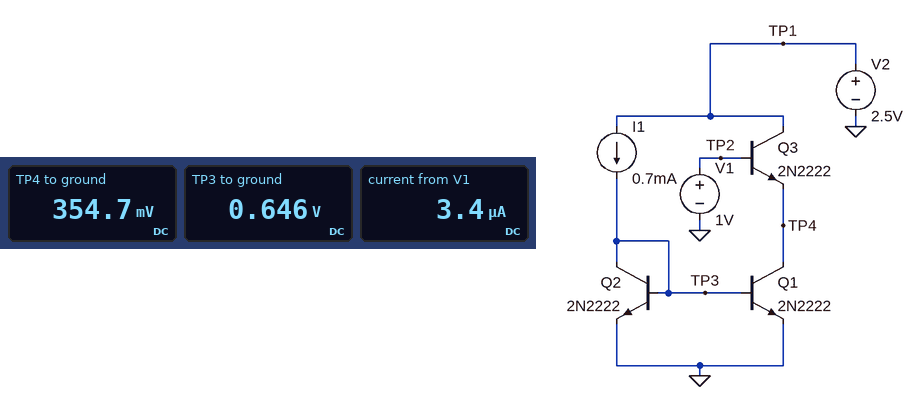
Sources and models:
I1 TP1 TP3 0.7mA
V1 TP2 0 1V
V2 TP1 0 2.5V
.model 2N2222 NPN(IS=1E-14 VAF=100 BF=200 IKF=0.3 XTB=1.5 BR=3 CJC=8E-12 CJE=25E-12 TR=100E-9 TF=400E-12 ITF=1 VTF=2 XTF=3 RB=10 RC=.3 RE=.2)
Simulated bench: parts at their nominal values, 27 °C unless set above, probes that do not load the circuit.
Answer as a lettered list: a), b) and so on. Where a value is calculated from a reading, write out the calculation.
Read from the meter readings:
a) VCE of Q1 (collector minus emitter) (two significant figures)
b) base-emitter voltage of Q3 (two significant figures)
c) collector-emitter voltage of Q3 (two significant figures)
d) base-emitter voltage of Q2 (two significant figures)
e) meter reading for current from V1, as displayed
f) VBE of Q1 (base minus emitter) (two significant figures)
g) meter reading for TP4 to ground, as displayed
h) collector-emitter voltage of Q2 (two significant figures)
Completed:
a) 354.7 mV = 350 mV
b) 1 V - 354.7 mV = 650 mV
c) 2.5 V - 354.7 mV = 2.1 V
d) 646 mV = 650 mV
e) 3.4 µA
f) 646 mV = 650 mV
g) 354.7 mV
h) 646 mV = 650 mV
